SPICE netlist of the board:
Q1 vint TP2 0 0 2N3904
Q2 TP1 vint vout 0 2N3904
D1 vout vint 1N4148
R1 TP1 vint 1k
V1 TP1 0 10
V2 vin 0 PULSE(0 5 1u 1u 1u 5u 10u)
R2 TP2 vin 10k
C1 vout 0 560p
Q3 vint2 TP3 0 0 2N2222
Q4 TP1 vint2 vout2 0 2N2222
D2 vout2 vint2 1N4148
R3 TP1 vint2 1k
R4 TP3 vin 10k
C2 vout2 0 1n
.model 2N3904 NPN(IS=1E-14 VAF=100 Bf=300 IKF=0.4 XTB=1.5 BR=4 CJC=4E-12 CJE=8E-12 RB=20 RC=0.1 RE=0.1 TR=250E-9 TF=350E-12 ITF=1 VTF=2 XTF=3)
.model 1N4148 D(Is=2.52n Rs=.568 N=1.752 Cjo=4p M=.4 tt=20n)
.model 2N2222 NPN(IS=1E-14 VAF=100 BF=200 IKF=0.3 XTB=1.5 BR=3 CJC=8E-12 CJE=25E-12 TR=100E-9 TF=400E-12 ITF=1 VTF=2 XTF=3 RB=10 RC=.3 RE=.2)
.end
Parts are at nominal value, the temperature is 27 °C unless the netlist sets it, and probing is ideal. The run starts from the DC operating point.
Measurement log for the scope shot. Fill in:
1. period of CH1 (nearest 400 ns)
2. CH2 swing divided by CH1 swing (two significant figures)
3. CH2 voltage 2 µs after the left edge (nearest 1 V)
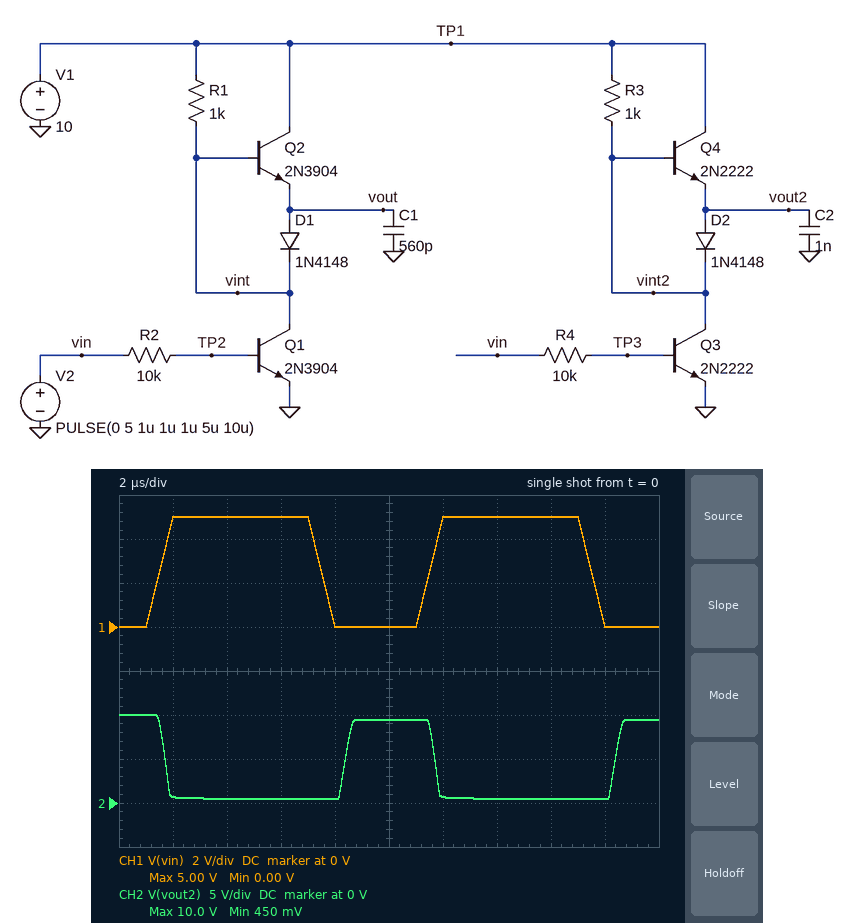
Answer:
10.0 µs
1.9
1 V
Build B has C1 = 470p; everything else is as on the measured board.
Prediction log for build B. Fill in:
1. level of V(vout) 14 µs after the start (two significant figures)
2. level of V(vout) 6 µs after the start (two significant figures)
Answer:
440 mV
410 mV
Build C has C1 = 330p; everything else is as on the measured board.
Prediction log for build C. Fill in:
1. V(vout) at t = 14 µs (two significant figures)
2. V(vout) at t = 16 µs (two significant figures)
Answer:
430 mV
390 mV
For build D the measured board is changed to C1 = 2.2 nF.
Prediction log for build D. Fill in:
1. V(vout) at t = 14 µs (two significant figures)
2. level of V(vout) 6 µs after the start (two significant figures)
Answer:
520 mV
480 mV
